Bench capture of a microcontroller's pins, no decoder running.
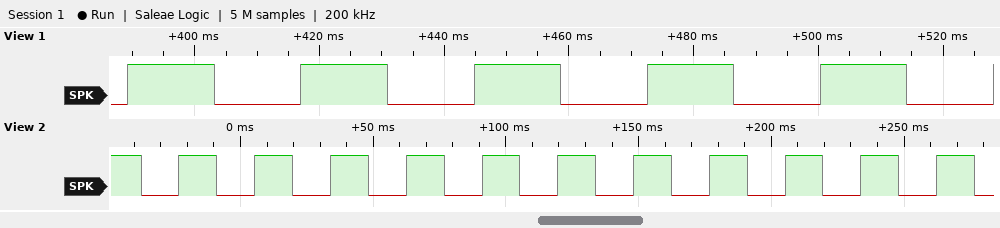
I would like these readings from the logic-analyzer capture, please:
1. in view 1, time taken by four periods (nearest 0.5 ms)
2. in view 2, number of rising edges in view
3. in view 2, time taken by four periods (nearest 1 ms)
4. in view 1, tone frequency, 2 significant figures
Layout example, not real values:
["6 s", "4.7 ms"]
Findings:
["111.0 ms", "11", "113 ms", "36 Hz"]
